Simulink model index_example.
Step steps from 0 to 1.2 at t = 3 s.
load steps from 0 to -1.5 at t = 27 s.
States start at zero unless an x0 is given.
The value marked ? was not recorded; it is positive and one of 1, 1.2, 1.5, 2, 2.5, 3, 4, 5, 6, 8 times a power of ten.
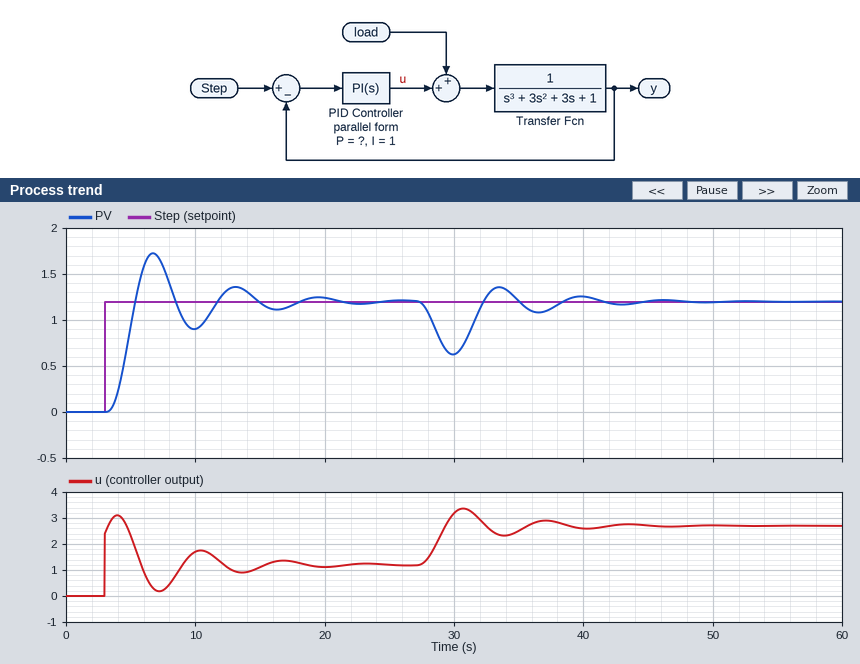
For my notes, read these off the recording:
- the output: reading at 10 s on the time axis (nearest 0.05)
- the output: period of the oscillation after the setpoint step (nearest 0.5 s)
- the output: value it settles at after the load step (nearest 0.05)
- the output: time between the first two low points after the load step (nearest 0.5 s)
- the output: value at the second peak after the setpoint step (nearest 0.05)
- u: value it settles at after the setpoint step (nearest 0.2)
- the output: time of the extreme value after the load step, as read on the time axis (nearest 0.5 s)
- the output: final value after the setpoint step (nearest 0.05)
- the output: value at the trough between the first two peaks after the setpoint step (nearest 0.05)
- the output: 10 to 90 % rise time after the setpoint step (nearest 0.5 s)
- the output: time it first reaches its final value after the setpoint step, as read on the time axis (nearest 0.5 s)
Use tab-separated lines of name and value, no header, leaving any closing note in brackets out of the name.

the output: reading at 10 s on the time axis	0.90
the output: period of the oscillation after the setpoint step	6.5 s
the output: value it settles at after the load step	1.20
the output: time between the first two low points after the load step	6.5 s
the output: value at the second peak after the setpoint step	1.35
u: value it settles at after the setpoint step	1.2
the output: time of the extreme value after the load step, as read on the time axis	30.0 s
the output: final value after the setpoint step	1.20
the output: value at the trough between the first two peaks after the setpoint step	0.90
the output: 10 to 90 % rise time after the setpoint step	1.5 s
the output: time it first reaches its final value after the setpoint step, as read on the time axis	5.5 s
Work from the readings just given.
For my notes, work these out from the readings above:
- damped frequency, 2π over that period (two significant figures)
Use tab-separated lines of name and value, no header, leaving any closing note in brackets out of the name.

damped frequency, 2π over that period	0.97 rad/s
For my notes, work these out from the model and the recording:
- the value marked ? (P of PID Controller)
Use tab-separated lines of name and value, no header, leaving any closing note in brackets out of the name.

the value marked ?	2
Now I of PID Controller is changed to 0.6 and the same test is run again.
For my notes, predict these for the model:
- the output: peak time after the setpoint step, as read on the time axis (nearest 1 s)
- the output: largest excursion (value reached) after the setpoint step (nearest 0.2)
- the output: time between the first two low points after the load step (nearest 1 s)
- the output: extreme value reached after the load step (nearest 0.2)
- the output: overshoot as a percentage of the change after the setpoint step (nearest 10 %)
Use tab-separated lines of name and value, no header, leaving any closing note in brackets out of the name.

the output: peak time after the setpoint step, as read on the time axis	7 s
the output: largest excursion (value reached) after the setpoint step	1.4
the output: time between the first two low points after the load step	6 s
the output: extreme value reached after the load step	0.6
the output: overshoot as a percentage of the change after the setpoint step	20 %
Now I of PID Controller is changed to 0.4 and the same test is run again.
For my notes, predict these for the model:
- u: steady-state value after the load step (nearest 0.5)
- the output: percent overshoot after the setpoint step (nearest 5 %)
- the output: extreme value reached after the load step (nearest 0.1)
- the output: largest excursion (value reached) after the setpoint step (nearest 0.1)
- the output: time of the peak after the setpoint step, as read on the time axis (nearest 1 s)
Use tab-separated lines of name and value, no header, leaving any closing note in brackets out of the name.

u: steady-state value after the load step	2.5
the output: percent overshoot after the setpoint step	10 %
the output: extreme value reached after the load step	0.6
the output: largest excursion (value reached) after the setpoint step	1.3
the output: time of the peak after the setpoint step, as read on the time axis	7 s
